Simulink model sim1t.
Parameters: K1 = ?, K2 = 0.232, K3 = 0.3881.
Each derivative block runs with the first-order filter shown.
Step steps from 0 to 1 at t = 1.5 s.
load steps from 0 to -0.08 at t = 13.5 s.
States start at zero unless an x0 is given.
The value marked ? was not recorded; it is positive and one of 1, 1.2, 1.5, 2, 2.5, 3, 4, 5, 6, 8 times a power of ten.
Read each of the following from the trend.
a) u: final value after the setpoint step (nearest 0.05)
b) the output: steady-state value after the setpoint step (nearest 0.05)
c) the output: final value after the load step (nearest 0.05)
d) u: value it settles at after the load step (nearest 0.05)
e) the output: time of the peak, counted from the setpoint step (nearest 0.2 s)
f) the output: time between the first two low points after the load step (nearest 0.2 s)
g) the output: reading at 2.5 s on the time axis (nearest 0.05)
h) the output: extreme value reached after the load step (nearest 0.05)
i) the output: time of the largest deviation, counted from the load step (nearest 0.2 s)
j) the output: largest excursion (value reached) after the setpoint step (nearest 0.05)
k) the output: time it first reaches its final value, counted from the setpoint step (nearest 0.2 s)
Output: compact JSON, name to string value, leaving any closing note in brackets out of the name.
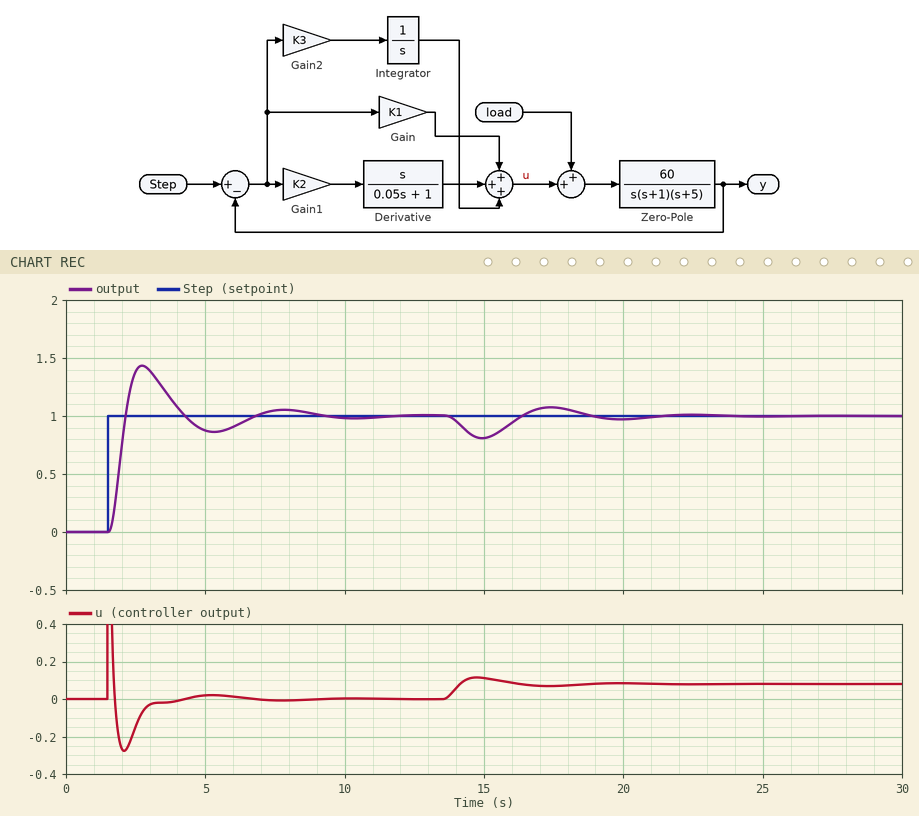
{"u: final value after the setpoint step": "0.00", "the output: steady-state value after the setpoint step": "1.00", "the output: final value after the load step": "1.00", "u: value it settles at after the load step": "0.10", "the output: time of the peak, counted from the setpoint step": "1.2 s", "the output: time between the first two low points after the load step": "5.0 s", "the output: reading at 2.5 s on the time axis": "1.40", "the output: extreme value reached after the load step": "0.80", "the output: time of the largest deviation, counted from the load step": "1.4 s", "the output: largest excursion (value reached) after the setpoint step": "1.45", "the output: time it first reaches its final value, counted from the setpoint step": "0.6 s"}
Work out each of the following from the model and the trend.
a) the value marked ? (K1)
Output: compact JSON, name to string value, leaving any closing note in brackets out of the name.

{"the value marked ?": "0.3"}
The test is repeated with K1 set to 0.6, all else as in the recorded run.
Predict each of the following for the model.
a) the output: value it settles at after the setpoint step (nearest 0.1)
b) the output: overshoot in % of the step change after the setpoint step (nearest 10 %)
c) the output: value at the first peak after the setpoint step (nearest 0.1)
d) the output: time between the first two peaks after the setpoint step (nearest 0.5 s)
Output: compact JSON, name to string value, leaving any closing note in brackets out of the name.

{"the output: value it settles at after the setpoint step": "1.0", "the output: overshoot in % of the step change after the setpoint step": "60 %", "the output: value at the first peak after the setpoint step": "1.6", "the output: time between the first two peaks after the setpoint step": "2.0 s"}
